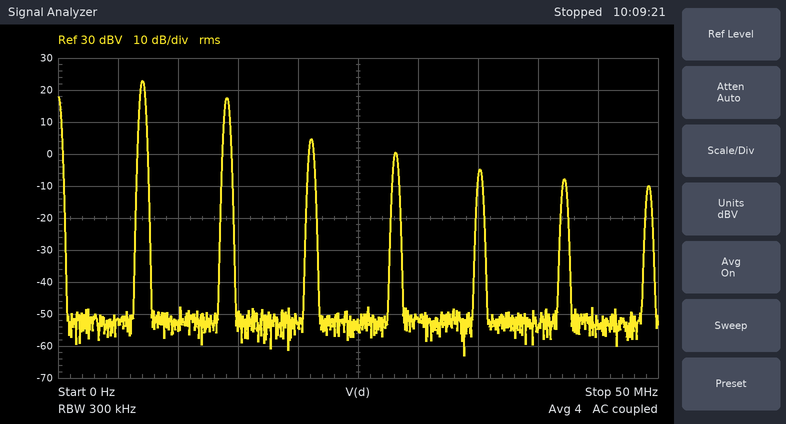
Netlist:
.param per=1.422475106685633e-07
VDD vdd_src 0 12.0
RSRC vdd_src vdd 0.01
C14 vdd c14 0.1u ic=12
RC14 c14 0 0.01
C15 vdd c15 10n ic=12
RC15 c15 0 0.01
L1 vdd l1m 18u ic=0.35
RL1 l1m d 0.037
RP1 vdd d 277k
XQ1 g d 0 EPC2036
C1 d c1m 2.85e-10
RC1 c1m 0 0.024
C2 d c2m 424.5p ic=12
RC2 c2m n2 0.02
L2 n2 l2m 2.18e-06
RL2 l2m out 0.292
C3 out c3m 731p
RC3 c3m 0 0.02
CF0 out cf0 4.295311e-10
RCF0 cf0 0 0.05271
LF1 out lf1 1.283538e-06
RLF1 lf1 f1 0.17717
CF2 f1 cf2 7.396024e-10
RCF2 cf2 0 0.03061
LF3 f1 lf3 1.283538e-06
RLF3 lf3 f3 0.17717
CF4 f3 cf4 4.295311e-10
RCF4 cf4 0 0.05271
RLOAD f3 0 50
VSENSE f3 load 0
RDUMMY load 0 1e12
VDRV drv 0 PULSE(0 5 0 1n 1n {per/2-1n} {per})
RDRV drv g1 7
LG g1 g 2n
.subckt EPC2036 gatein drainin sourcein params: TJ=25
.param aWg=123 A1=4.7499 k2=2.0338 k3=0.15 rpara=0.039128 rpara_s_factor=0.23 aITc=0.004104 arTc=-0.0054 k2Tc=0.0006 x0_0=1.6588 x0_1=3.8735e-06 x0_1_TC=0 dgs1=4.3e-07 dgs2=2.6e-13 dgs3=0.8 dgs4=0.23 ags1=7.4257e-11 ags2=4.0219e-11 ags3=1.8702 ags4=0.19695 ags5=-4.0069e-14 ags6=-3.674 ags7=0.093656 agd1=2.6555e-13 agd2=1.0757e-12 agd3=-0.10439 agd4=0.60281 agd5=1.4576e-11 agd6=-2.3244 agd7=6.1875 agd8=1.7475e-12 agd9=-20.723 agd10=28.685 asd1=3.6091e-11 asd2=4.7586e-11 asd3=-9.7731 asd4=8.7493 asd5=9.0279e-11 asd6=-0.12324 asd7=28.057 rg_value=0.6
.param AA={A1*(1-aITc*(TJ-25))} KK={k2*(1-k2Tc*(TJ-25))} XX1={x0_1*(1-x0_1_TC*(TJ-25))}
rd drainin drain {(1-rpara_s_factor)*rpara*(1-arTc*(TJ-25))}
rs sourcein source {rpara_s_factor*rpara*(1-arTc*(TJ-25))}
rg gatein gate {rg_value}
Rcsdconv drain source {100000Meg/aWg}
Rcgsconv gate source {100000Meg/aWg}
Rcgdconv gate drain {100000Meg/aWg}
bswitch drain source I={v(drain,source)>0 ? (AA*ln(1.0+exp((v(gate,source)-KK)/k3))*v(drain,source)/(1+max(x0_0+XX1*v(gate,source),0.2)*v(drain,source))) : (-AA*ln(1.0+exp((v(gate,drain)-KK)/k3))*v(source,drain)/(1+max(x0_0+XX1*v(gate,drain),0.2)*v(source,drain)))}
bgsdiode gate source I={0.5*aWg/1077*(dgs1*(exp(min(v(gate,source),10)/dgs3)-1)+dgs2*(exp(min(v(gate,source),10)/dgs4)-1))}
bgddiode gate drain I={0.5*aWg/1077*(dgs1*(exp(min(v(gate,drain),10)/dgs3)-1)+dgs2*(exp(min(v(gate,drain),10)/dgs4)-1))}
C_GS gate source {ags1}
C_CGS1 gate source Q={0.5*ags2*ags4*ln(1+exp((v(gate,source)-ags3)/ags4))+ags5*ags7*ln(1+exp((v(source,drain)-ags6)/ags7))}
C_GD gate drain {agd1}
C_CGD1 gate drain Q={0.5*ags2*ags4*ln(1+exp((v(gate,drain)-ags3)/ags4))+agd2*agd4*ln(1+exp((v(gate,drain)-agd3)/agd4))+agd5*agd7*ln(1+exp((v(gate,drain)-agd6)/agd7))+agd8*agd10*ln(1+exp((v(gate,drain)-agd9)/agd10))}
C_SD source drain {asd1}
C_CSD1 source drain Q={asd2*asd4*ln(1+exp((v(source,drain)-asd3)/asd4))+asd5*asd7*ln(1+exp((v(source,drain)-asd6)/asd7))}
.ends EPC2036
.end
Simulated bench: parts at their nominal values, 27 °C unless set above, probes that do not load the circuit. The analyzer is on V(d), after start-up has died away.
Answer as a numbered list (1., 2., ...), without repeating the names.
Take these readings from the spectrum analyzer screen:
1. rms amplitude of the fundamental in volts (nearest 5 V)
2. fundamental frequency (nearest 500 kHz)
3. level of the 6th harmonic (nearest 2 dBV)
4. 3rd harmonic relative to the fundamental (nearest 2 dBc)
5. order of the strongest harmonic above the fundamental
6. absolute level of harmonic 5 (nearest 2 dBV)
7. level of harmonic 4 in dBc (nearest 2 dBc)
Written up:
1. 15 V
2. 7.0 MHz
3. -8 dBV
4. -18 dBc
5. 2
6. -4 dBV
7. -22 dBc
